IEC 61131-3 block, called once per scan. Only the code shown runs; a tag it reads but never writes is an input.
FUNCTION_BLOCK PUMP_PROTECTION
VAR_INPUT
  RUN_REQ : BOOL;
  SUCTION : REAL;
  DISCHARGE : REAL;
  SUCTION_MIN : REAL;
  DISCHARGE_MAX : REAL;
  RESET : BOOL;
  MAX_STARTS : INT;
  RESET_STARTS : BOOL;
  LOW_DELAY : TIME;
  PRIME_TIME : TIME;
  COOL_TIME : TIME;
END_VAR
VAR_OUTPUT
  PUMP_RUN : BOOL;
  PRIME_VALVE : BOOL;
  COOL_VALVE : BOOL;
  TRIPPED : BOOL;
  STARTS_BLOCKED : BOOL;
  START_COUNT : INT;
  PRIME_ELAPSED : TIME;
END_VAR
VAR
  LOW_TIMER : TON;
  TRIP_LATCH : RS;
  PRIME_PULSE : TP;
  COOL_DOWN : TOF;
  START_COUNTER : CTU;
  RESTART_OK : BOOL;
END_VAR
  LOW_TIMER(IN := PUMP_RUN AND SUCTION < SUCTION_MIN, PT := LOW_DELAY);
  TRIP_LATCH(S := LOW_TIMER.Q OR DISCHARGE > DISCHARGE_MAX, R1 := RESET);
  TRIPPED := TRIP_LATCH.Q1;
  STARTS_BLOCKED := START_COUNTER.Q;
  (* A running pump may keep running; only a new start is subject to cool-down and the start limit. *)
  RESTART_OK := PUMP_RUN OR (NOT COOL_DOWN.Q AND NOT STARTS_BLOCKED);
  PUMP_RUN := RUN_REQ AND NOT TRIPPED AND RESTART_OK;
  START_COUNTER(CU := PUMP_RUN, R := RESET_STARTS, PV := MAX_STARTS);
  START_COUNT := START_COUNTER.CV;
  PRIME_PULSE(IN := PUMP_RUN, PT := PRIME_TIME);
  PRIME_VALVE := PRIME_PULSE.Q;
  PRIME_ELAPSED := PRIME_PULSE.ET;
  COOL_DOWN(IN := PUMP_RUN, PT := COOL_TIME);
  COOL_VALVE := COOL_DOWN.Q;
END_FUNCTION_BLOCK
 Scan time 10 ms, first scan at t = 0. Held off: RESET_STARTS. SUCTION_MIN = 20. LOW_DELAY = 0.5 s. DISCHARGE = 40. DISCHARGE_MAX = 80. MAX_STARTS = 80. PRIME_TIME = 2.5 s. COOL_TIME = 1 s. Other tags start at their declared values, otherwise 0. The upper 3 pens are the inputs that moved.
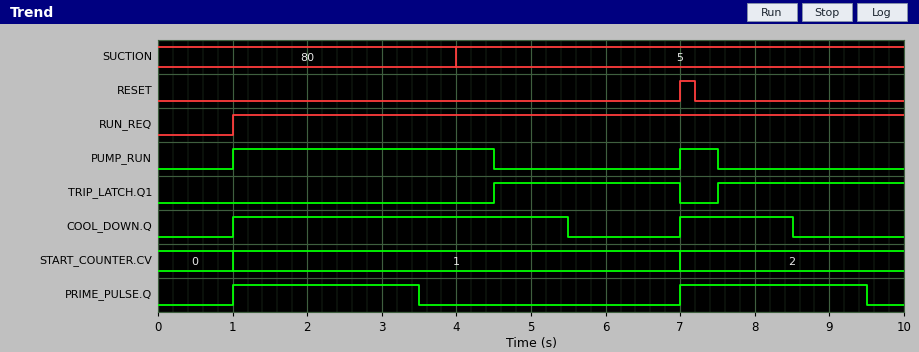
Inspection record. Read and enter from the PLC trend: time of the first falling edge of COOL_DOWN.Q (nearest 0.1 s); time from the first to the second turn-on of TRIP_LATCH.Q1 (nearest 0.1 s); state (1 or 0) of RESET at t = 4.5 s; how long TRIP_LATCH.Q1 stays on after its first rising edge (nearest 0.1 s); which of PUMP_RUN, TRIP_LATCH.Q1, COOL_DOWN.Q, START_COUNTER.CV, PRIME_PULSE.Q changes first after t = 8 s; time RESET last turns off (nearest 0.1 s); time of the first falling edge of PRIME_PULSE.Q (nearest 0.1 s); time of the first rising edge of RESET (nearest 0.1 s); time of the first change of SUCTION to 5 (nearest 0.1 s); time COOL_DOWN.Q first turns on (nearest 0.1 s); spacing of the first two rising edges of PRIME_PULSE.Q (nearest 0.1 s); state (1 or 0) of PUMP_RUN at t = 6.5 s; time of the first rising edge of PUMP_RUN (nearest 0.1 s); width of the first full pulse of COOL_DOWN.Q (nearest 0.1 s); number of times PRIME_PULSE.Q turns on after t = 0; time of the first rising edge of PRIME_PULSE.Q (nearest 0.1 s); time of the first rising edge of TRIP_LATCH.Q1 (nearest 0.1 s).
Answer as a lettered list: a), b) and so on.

a) 5.5 s
b) 3.0 s
c) 0
d) 2.5 s
e) COOL_DOWN.Q
f) 7.2 s
g) 3.5 s
h) 7.0 s
i) 4.0 s
j) 1.0 s
k) 6.0 s
l) 0
m) 1.0 s
n) 4.5 s
o) 2
p) 1.0 s
q) 4.5 s
